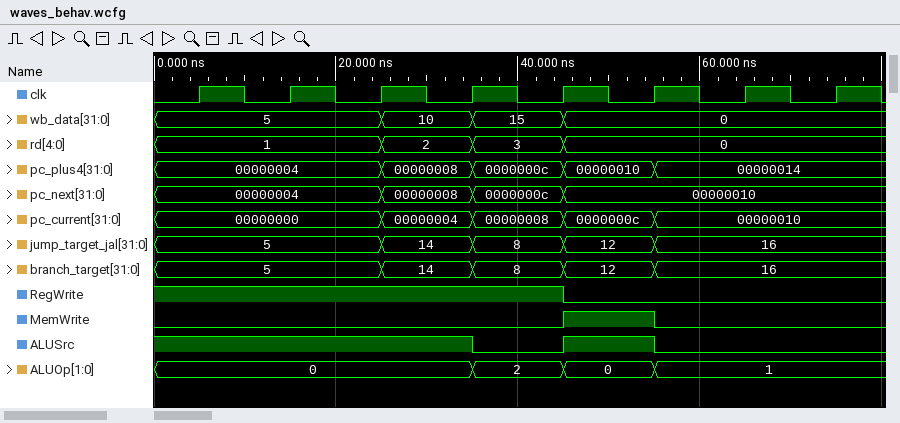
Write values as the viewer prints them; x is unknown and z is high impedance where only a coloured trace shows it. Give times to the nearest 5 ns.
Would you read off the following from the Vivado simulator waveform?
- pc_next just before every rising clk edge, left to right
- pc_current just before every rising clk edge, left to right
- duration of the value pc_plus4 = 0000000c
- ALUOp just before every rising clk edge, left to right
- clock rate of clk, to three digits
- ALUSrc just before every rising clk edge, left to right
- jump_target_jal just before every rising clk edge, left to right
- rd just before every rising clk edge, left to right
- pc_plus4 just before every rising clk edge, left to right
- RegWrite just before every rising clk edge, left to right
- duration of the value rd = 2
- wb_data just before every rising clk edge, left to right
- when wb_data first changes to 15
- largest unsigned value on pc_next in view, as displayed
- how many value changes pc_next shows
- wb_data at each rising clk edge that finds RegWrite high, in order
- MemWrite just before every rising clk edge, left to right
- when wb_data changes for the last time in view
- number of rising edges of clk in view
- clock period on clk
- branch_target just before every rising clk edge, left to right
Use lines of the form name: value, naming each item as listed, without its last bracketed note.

pc_next just before every rising clk edge, left to right: 00000004, 00000004, 00000004, 00000008, 0000000c, 00000010, 00000010, 00000010
pc_current just before every rising clk edge, left to right: 00000000, 00000000, 00000000, 00000004, 00000008, 0000000c, 00000010, 00000010
duration of the value pc_plus4 = 0000000c: 10 ns
ALUOp just before every rising clk edge, left to right: 0, 0, 0, 0, 2, 0, 1, 1
clock rate of clk, to three digits: 100 MHz
ALUSrc just before every rising clk edge, left to right: 1 1 1 1 0 1 0 0
jump_target_jal just before every rising clk edge, left to right: 5, 5, 5, 14, 8, 12, 16, 16
rd just before every rising clk edge, left to right: 1, 1, 1, 2, 3, 0, 0, 0
pc_plus4 just before every rising clk edge, left to right: 00000004, 00000004, 00000004, 00000008, 0000000c, 00000010, 00000014, 00000014
RegWrite just before every rising clk edge, left to right: 1 1 1 1 1 0 0 0
duration of the value rd = 2: 10 ns
wb_data just before every rising clk edge, left to right: 5, 5, 5, 10, 15, 0, 0, 0
when wb_data first changes to 15: 35 ns
largest unsigned value on pc_next in view, as displayed: 00000010
how many value changes pc_next shows: 3
wb_data at each rising clk edge that finds RegWrite high, in order: 5, 5, 5, 10, 15
MemWrite just before every rising clk edge, left to right: 0 0 0 0 0 1 0 0
when wb_data changes for the last time in view: 45 ns
number of rising edges of clk in view: 8
clock period on clk: 10 ns
branch_target just before every rising clk edge, left to right: 5, 5, 5, 14, 8, 12, 16, 16
